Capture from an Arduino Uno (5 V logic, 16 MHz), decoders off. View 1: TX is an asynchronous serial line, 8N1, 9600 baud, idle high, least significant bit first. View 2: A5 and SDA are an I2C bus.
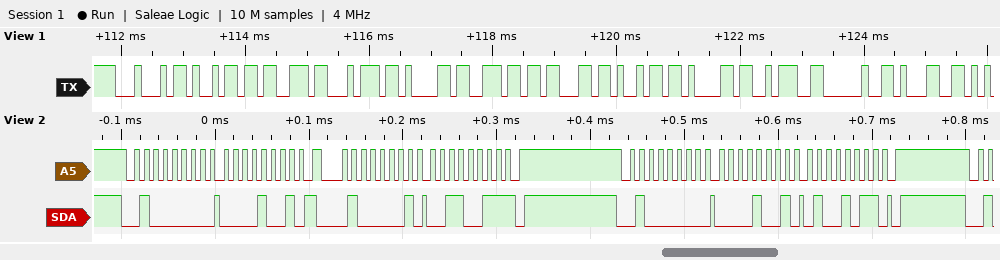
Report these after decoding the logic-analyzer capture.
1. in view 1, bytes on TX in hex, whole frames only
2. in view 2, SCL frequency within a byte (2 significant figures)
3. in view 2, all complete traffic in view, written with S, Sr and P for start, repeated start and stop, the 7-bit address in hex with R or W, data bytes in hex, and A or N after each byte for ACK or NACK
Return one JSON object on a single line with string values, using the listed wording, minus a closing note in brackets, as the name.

{"in view 1, bytes on TX in hex, whole frames only": "44 69 73 74 61 6E 63 69 61 3A 20 31", "in view 2, SCL frequency within a byte": "100 kHz", "in view 2, all complete traffic in view, written with S, Sr and P for start, repeated start and stop, the 7-bit address in hex with R or W, data bytes in hex, and A or N after each byte for ACK or NACK": "S 20W A 09 A Sr 20R A 33 N P S 20W A 09 A 4B A P"}
